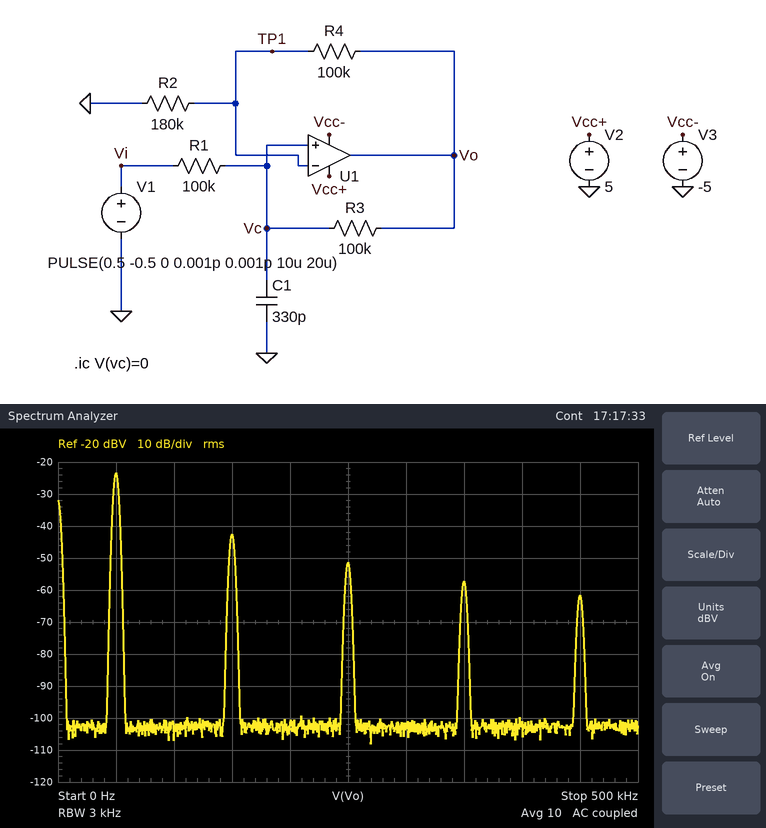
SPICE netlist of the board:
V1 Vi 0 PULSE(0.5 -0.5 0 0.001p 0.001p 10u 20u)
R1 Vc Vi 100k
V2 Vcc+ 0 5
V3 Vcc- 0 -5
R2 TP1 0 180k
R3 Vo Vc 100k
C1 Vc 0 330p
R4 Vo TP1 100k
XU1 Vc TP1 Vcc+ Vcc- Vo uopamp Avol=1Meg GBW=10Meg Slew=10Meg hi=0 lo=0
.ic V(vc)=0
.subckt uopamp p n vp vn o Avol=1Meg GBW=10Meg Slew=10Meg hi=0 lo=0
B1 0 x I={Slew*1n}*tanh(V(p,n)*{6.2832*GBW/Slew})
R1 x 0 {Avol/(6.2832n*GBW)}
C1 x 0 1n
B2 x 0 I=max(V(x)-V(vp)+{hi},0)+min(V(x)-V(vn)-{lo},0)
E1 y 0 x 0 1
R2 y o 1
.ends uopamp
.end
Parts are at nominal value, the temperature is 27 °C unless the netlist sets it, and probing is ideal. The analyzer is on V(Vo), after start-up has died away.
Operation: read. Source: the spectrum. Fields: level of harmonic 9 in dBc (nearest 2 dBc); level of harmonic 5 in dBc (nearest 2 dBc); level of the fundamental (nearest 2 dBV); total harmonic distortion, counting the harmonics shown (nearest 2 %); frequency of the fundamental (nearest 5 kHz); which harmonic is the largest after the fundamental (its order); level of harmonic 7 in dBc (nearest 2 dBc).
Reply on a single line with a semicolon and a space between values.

-38 dBc; -28 dBc; -24 dBV; 12 %; 50 kHz; 3; -34 dBc
